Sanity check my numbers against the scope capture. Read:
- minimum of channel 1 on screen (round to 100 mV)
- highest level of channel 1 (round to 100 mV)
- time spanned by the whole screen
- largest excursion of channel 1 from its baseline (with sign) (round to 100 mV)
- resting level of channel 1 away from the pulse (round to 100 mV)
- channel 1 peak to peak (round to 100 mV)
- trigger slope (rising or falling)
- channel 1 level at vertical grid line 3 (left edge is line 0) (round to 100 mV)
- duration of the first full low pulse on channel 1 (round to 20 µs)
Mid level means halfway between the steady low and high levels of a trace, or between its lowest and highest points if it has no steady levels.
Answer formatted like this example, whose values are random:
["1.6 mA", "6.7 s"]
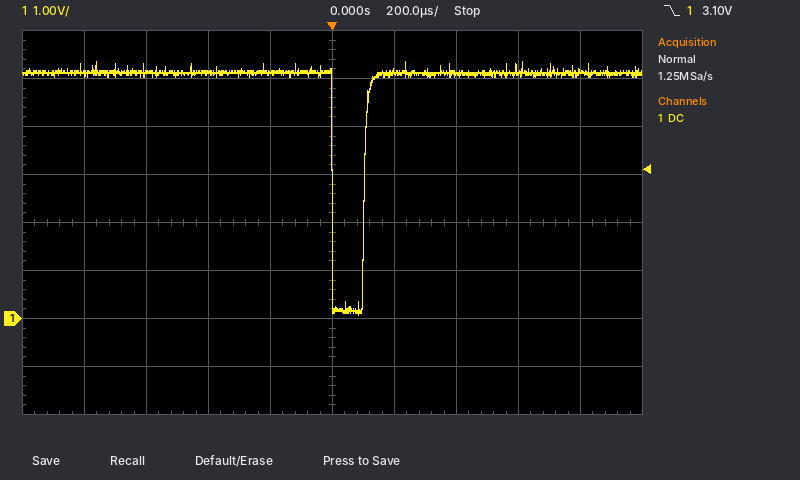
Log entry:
["100 mV", "5.4 V", "2 ms", "-5.0 V", "5.1 V", "5.3 V", "falling", "5.1 V", "100 µs"]
